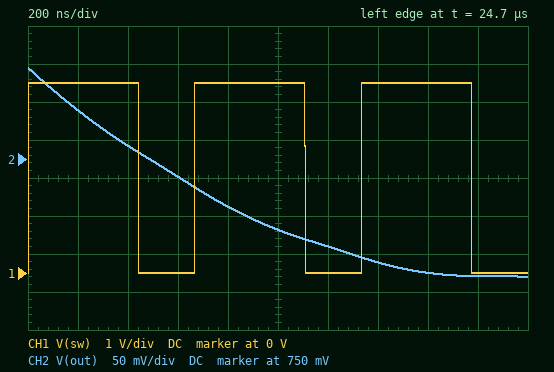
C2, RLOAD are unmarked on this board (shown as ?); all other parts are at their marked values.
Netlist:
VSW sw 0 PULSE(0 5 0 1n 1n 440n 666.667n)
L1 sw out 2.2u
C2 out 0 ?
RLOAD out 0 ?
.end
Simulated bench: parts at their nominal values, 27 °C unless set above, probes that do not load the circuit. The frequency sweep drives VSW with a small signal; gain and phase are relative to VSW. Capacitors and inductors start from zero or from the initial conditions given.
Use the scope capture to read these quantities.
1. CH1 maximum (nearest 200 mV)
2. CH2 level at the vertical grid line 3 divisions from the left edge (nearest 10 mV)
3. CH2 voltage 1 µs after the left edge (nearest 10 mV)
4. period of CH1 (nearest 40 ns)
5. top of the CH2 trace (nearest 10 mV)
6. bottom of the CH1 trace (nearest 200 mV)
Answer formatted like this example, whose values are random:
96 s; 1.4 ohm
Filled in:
5.0 V; 730 mV; 660 mV; 680 ns; 870 mV; 0 V
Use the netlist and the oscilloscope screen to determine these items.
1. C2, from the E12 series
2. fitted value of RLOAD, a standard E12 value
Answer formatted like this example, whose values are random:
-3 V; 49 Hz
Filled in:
8.2 µF; 8.2 Ω
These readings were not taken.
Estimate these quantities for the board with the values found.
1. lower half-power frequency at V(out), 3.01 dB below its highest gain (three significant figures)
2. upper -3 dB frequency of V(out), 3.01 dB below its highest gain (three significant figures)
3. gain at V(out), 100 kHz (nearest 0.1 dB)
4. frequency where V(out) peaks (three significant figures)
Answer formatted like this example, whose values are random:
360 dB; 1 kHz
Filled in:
36.2 kHz; 38.6 kHz; -15.7 dB; 37.4 kHz
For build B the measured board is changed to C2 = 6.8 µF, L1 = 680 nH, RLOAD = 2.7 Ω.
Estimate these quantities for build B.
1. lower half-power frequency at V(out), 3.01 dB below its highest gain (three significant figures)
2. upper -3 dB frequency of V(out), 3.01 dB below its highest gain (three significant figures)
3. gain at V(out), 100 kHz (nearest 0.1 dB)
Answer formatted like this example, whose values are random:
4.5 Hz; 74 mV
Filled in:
69.3 kHz; 78.0 kHz; 1.5 dB
